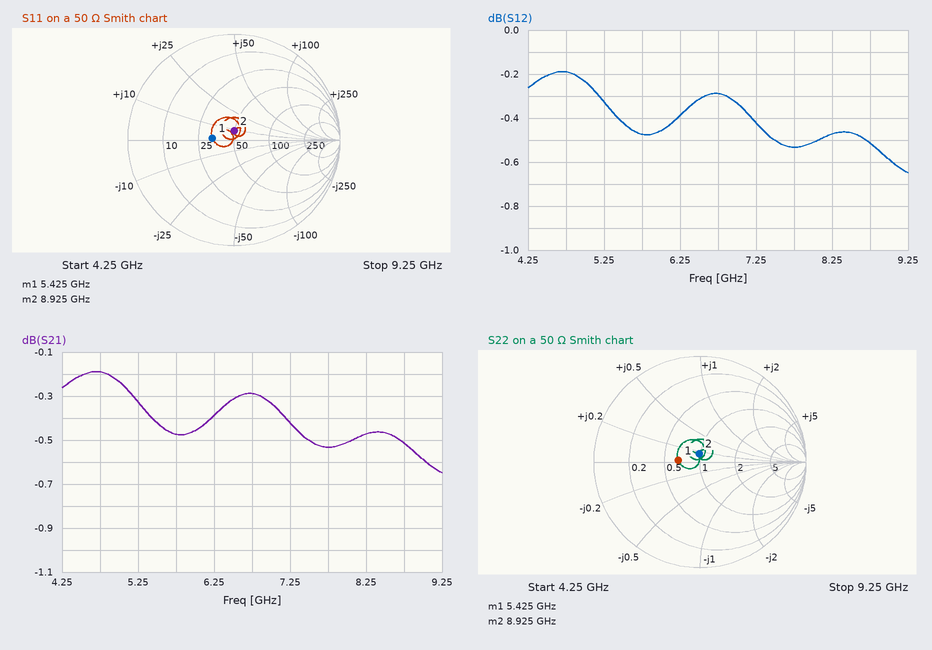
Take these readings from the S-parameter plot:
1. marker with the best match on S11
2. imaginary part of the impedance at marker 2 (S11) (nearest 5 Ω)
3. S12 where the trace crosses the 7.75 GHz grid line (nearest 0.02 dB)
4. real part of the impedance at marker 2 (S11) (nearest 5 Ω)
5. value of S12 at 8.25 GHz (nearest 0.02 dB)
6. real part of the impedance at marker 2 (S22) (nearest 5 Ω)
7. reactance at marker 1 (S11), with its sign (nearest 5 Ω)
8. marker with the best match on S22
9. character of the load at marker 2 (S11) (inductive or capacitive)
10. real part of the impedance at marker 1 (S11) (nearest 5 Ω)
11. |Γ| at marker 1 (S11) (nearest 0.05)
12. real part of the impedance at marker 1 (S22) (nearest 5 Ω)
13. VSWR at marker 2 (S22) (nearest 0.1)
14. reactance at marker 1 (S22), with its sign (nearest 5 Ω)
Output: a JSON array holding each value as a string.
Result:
["marker 2", "+10 Ω", "-0.54 dB", "50 Ω", "-0.48 dB", "50 Ω", "0 Ω", "marker 2", "inductive", "35 Ω", "0.20", "35 Ω", "1.2", "0 Ω"]
